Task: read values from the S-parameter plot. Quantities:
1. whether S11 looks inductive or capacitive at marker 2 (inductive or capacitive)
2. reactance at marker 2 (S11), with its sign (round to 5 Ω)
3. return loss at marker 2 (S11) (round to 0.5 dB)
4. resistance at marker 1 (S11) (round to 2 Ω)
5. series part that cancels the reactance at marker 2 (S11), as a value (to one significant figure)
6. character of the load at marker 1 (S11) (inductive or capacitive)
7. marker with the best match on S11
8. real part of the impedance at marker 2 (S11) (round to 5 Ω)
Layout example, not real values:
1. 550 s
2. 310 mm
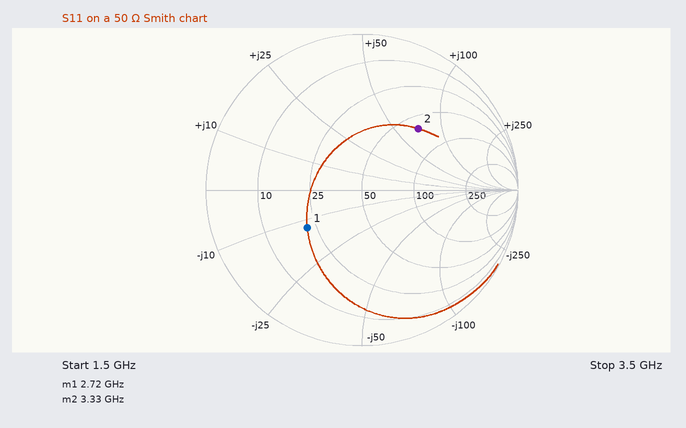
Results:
1. inductive
2. +70 Ω
3. 5.5 dB
4. 22 Ω
5. 700 fF
6. capacitive
7. marker 1
8. 65 Ω
